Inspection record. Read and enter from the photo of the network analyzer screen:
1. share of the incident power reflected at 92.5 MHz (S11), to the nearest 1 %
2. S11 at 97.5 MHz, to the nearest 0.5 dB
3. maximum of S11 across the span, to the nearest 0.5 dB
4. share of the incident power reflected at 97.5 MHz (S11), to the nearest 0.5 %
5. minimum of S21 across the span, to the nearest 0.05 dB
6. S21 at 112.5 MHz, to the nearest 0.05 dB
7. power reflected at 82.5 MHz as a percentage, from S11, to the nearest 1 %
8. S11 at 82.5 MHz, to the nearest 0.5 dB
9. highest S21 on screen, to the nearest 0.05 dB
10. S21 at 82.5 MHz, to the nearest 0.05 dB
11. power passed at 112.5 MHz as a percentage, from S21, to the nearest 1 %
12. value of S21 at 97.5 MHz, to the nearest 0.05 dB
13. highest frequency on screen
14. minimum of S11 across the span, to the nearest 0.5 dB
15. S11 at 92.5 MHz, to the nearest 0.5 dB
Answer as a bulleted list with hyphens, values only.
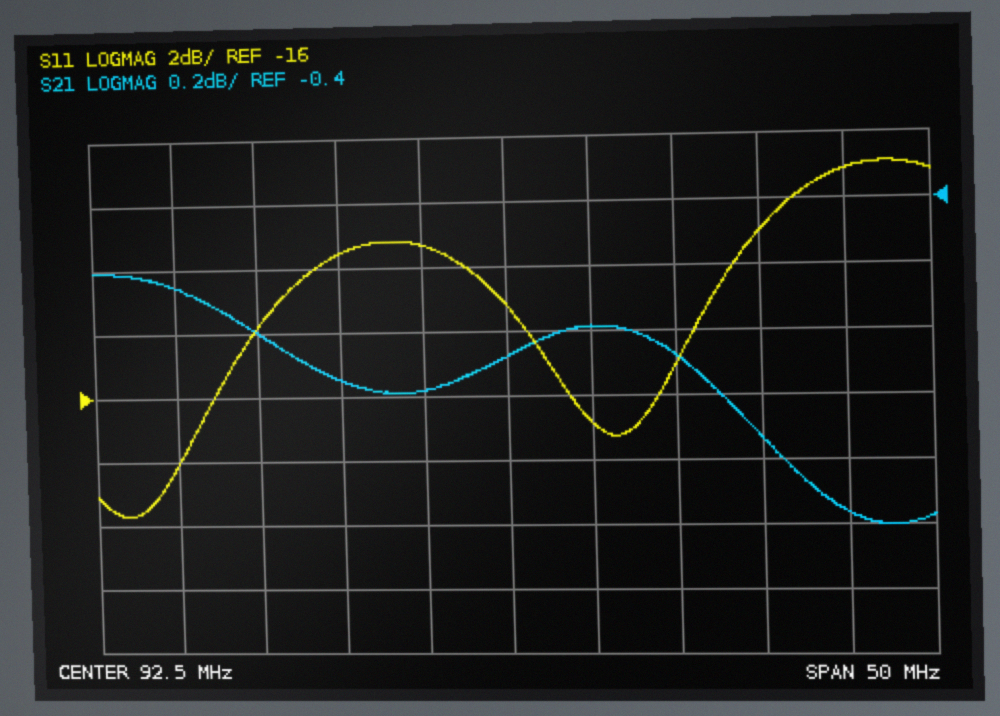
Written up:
- 5 %
- -17.0 dB
- -9.0 dB
- 2.0 %
- -1.40 dB
- -1.35 dB
- 7 %
- -11.5 dB
- -0.60 dB
- -0.95 dB
- 73 %
- -0.80 dB
- 117.5 MHz
- -19.5 dB
- -13.0 dB
